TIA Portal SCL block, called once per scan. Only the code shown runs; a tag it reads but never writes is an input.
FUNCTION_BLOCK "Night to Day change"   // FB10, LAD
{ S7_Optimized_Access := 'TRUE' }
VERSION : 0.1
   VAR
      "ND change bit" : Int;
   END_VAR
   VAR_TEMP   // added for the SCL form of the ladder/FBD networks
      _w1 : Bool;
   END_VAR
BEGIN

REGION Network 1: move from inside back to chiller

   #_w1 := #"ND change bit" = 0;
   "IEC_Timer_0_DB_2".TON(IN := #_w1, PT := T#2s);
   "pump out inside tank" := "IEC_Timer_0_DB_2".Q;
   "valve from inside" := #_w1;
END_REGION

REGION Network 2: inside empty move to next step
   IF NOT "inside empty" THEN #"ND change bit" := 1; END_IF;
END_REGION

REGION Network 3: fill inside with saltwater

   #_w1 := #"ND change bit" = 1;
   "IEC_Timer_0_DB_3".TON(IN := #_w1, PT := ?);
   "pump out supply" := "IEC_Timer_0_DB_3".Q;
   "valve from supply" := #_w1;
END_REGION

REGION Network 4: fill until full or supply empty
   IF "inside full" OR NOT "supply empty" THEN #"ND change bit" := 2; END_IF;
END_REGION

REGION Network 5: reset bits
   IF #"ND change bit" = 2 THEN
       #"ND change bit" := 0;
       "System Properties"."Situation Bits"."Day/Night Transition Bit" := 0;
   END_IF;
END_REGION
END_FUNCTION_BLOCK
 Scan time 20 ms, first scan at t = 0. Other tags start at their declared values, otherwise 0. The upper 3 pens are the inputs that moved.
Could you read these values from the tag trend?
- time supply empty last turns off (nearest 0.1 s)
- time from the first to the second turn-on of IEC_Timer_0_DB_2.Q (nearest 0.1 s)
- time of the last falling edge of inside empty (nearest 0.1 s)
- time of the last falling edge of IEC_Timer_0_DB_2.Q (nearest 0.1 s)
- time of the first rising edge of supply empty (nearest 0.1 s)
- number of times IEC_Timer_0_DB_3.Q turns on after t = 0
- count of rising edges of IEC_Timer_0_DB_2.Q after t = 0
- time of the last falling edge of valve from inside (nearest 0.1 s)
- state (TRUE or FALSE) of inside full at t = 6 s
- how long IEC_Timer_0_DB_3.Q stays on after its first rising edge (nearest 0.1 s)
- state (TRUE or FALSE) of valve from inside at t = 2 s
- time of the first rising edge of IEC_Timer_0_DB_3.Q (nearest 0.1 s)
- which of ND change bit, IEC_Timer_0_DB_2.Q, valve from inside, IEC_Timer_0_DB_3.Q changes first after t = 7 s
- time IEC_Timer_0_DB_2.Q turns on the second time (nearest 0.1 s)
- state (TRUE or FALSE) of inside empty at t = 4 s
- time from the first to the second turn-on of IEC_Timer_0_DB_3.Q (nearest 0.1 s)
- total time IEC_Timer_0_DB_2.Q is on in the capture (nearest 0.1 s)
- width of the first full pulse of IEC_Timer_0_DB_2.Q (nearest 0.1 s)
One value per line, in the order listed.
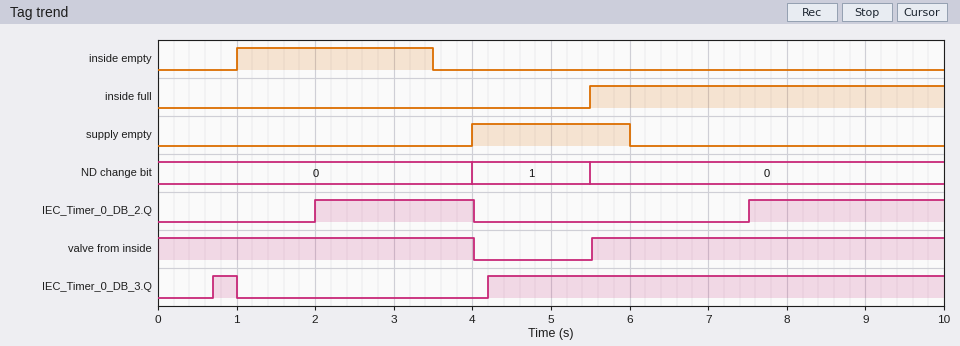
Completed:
6.0 s
5.5 s
3.5 s
4.0 s
4.0 s
2
2
4.0 s
TRUE
0.3 s
TRUE
0.7 s
IEC_Timer_0_DB_2.Q
7.5 s
FALSE
3.5 s
4.5 s
2.0 s
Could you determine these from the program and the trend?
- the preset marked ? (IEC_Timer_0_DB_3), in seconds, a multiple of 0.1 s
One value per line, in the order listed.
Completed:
0.7 s
